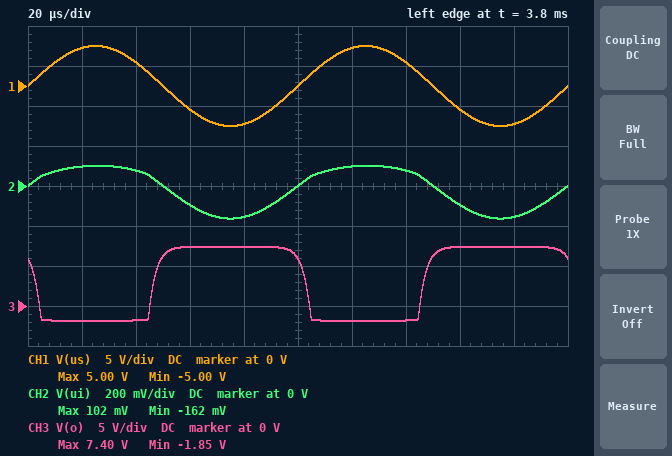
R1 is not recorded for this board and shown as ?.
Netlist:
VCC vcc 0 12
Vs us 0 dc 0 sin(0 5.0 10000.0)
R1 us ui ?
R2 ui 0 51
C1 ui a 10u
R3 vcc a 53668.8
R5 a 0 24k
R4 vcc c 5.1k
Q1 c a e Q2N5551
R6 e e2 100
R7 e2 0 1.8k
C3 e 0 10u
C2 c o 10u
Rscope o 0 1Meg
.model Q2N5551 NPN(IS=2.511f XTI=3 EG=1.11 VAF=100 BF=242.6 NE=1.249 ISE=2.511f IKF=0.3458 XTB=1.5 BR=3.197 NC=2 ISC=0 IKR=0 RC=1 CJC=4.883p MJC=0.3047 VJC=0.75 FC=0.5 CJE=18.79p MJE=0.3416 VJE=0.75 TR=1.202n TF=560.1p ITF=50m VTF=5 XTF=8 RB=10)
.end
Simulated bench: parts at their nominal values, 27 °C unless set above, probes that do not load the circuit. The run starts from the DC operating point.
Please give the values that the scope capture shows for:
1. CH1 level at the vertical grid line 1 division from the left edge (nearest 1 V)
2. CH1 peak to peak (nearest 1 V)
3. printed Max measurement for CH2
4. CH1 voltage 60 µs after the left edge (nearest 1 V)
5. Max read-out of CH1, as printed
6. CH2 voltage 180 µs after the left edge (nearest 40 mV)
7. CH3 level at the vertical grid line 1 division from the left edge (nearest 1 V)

5 V
10 V
102 mV
-3 V
5.00 V
-160 mV
-2 V
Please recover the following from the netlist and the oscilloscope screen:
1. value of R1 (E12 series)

1.5 kΩ
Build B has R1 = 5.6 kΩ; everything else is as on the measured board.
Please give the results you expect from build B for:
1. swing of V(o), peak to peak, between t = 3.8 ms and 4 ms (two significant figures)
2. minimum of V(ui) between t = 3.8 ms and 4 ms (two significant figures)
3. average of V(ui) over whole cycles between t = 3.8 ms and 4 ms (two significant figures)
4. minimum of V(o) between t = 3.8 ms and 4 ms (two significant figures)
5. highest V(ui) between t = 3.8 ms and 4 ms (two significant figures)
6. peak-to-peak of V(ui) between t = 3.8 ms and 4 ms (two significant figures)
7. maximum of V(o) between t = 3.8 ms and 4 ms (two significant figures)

7.7 V
-44 mV
-5.6 mV
-1.8 V
25 mV
69 mV
5.9 V
